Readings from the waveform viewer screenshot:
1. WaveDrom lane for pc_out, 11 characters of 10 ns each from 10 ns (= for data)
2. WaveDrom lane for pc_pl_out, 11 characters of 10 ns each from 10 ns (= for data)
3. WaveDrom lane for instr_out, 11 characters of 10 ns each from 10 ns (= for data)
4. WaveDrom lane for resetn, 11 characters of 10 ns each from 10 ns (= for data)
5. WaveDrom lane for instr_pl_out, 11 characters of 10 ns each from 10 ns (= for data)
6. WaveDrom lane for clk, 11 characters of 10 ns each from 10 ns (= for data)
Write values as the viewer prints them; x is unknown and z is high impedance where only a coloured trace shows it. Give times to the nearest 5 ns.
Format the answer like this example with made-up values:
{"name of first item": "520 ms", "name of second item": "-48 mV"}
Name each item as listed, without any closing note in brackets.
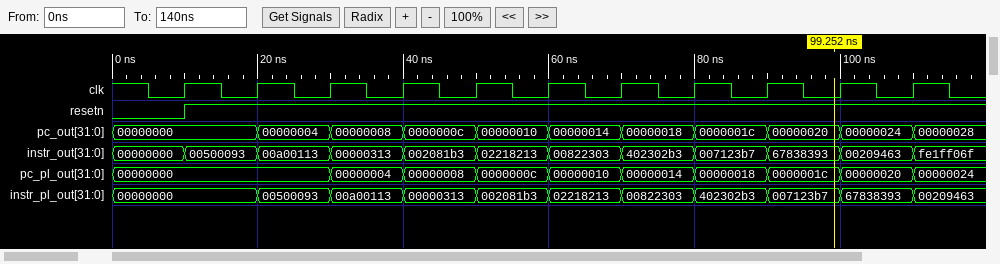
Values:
{"WaveDrom lane for pc_out, 11 characters of 10 ns each from 10 ns": "{name: 'pc_out', wave: '===========', data: '00000000 00000004 00000008 0000000c 00000010 00000014 00000018 0000001c 00000020 00000024 00000028'}", "WaveDrom lane for pc_pl_out, 11 characters of 10 ns each from 10 ns": "{name: 'pc_pl_out', wave: '=.=========', data: '00000000 00000004 00000008 0000000c 00000010 00000014 00000018 0000001c 00000020 00000024'}", "WaveDrom lane for instr_out, 11 characters of 10 ns each from 10 ns": "{name: 'instr_out', wave: '===========', data: '00500093 00a00113 00000313 002081b3 02218213 00822303 402302b3 007123b7 67838393 00209463 fe1ff06f'}", "WaveDrom lane for resetn, 11 characters of 10 ns each from 10 ns": "{name: 'resetn', wave: '1..........'}", "WaveDrom lane for instr_pl_out, 11 characters of 10 ns each from 10 ns": "{name: 'instr_pl_out', wave: '===========', data: '00000000 00500093 00a00113 00000313 002081b3 02218213 00822303 402302b3 007123b7 67838393 00209463'}", "WaveDrom lane for clk, 11 characters of 10 ns each from 10 ns": "{name: 'clk', wave: 'p..........'}"}
